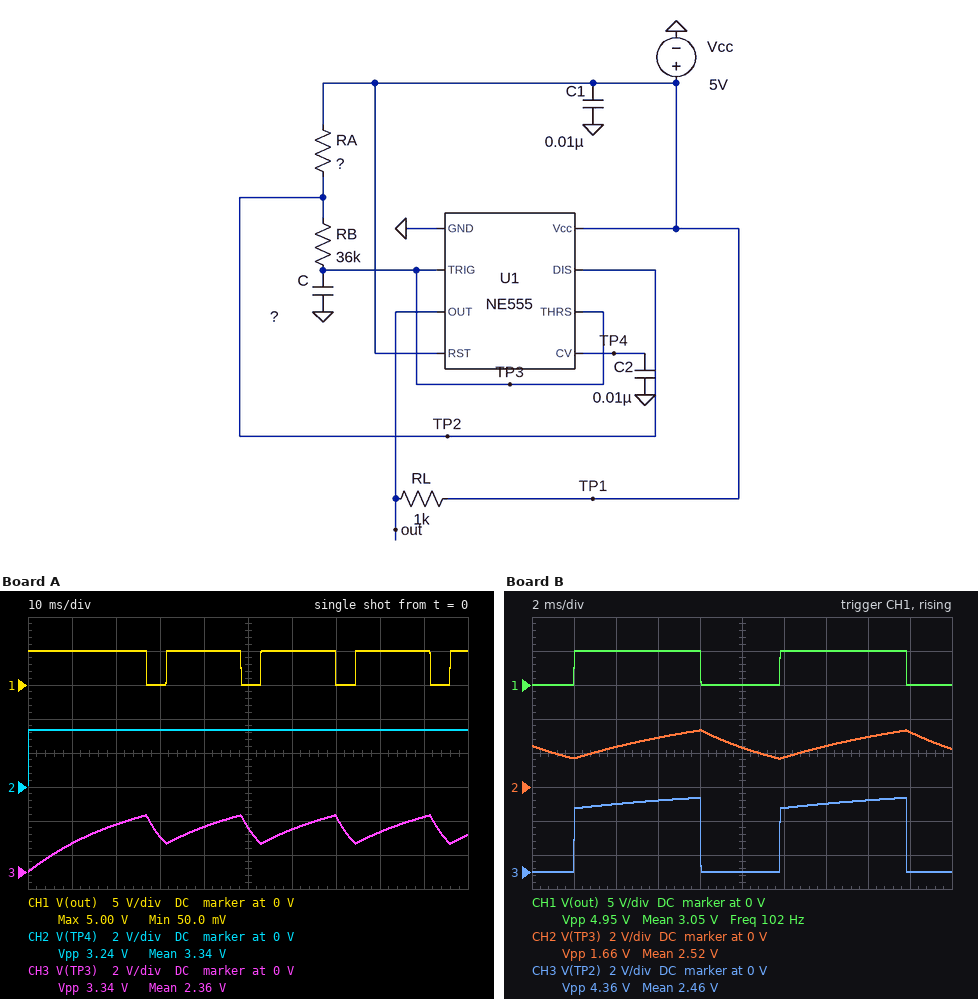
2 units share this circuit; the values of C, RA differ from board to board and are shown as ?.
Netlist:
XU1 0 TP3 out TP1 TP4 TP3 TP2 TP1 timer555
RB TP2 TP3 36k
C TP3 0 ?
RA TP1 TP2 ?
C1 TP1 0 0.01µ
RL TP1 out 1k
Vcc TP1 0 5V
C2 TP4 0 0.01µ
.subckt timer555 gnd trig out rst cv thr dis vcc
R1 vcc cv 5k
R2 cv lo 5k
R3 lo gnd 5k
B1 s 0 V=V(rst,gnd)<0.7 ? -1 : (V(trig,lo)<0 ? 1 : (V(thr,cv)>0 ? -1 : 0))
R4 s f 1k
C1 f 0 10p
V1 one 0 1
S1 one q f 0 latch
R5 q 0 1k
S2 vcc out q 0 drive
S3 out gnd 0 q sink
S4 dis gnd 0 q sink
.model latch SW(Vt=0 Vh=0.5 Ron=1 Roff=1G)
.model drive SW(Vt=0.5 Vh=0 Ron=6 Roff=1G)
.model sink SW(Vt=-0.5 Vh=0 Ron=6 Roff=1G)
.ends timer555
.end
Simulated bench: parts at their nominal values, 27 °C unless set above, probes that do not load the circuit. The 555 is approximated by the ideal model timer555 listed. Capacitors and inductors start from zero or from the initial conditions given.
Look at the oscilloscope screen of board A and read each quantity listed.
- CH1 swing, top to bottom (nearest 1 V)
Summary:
5 V
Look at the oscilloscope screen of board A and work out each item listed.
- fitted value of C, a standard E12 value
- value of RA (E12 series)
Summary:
180 nF
100 kΩ
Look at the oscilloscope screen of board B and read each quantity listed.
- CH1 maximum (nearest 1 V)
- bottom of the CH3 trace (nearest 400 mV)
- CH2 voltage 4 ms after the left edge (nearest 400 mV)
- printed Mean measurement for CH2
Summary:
5 V
0 V
2.4 V
2.52 V
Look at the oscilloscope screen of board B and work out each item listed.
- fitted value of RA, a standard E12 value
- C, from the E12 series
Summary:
22 kΩ
150 nF
